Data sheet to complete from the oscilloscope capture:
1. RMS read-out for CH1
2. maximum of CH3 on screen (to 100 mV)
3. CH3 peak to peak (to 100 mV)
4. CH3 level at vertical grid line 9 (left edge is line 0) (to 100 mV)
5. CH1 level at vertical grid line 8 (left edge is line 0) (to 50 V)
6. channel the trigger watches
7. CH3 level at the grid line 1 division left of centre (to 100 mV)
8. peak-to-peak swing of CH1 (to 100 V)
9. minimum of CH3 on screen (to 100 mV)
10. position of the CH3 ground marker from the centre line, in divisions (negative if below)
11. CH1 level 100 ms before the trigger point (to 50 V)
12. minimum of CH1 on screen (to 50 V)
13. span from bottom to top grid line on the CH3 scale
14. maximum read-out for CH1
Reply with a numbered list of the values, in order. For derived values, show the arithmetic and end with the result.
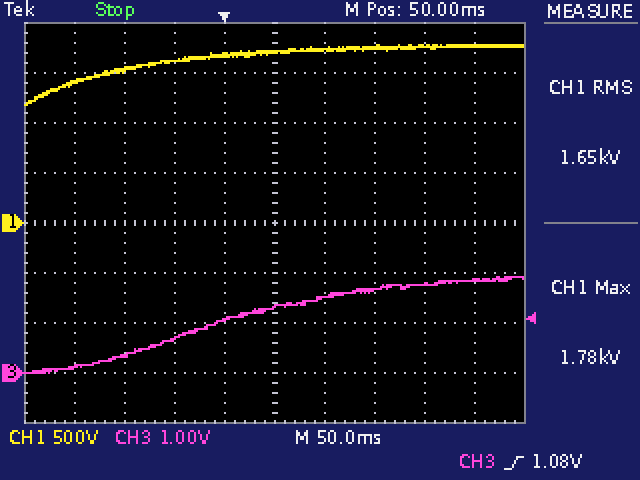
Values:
1. 1.65 kV
2. 1.9 V
3. 1.9 V − (0.0 V) = 1.9 V
4. 1.9 V
5. 1.75 kV
6. CH3
7. 1.1 V
8. 600 V
9. 0.0 V
10. -3.0 div
11. 1.55 kV
12. 1.20 kV
13. 8 V
14. 1.78 kV
